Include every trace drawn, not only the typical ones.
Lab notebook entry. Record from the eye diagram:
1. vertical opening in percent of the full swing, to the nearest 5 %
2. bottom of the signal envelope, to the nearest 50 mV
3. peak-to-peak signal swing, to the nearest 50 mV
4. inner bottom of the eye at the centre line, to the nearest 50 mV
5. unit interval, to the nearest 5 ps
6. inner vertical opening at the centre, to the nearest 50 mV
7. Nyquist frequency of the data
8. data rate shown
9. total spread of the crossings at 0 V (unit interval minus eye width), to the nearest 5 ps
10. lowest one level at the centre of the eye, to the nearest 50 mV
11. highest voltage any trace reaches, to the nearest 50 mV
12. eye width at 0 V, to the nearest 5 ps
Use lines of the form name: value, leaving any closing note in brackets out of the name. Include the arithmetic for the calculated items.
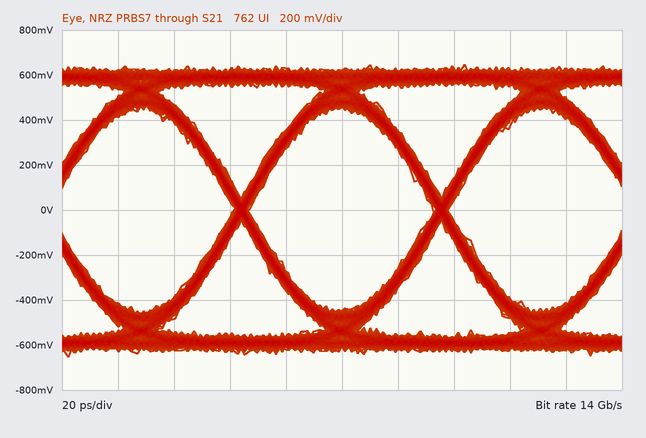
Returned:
vertical opening in percent of the full swing, to the nearest 5 %: 900 mV / 1.30 V ≈ 69.2 %, so 70 % to the nearest 5 %
bottom of the signal envelope, to the nearest 50 mV: -650 mV
peak-to-peak signal swing, to the nearest 50 mV: 1.30 V
inner bottom of the eye at the centre line, to the nearest 50 mV: -450 mV
unit interval, to the nearest 5 ps: 70 ps
inner vertical opening at the centre, to the nearest 50 mV: 900 mV
Nyquist frequency of the data: 7 GHz
data rate shown: 14 Gb/s
total spread of the crossings at 0 V (unit interval minus eye width), to the nearest 5 ps: 5 ps
lowest one level at the centre of the eye, to the nearest 50 mV: 450 mV
highest voltage any trace reaches, to the nearest 50 mV: 650 mV
eye width at 0 V, to the nearest 5 ps: 65 ps
